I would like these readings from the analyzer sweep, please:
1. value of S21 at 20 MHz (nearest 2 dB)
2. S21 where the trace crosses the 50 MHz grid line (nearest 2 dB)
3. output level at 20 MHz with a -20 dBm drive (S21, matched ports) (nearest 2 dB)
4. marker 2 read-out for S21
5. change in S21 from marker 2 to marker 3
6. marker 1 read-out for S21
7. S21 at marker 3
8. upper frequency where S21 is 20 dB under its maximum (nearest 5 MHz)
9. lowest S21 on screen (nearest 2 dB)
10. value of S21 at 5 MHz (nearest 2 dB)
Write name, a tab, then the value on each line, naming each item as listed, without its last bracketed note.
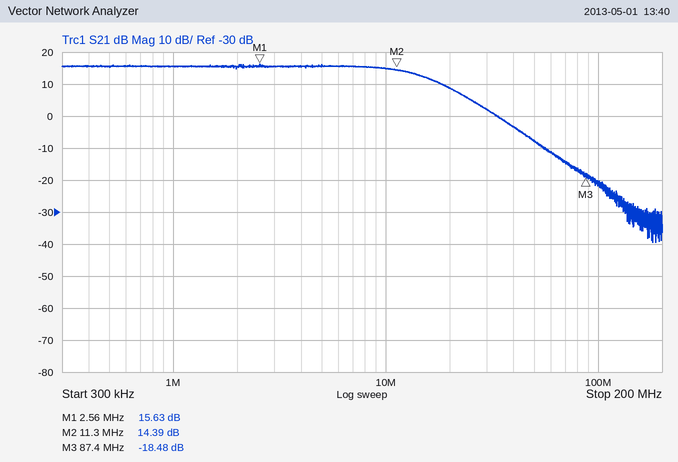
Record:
value of S21 at 20 MHz	8 dB
S21 where the trace crosses the 50 MHz grid line	-8 dB
output level at 20 MHz with a -20 dBm drive (S21, matched ports)	-12 dBm
marker 2 read-out for S21	14.39 dB
change in S21 from marker 2 to marker 3	-32.87 dB
marker 1 read-out for S21	15.63 dB
S21 at marker 3	-18.48 dB
upper frequency where S21 is 20 dB under its maximum	40 MHz
lowest S21 on screen	-40 dB
value of S21 at 5 MHz	16 dB
